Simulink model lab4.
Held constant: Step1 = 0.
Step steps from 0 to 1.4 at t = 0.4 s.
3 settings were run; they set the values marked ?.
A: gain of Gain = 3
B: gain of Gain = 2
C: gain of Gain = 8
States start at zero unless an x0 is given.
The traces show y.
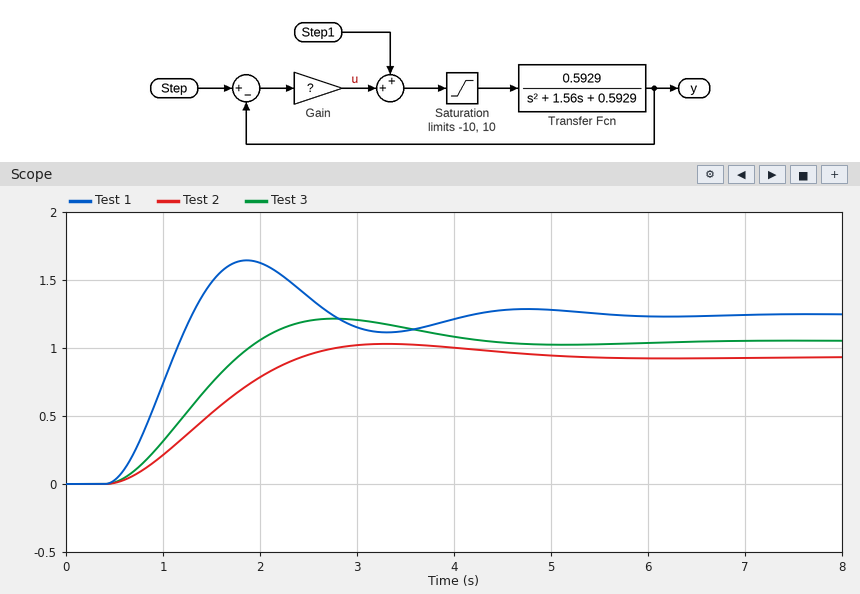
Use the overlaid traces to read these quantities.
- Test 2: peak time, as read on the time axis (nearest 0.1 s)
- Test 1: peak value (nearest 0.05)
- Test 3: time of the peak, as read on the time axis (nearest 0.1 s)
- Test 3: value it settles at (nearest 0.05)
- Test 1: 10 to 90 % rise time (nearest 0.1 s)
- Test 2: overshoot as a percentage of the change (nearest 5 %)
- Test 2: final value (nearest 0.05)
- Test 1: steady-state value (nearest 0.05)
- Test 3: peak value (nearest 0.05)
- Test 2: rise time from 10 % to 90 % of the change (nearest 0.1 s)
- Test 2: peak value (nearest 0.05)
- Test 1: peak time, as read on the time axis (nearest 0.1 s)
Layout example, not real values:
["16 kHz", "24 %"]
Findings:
["3.3 s", "1.65", "2.8 s", "1.05", "0.6 s", "10 %", "0.95", "1.25", "1.20", "1.4 s", "1.05", "1.9 s"]
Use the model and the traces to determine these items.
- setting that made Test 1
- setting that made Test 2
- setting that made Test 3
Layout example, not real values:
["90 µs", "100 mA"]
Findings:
["C", "B", "A"]
